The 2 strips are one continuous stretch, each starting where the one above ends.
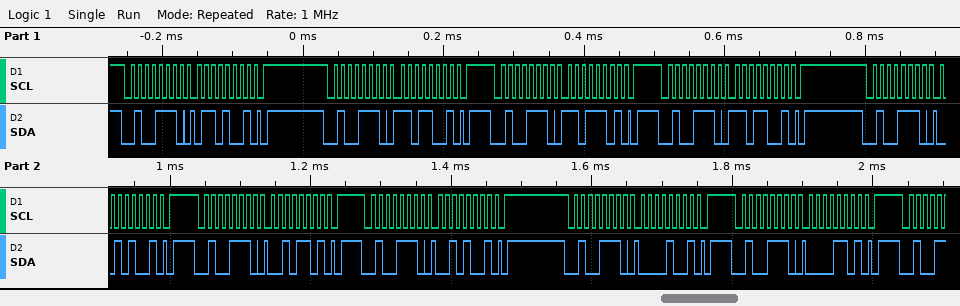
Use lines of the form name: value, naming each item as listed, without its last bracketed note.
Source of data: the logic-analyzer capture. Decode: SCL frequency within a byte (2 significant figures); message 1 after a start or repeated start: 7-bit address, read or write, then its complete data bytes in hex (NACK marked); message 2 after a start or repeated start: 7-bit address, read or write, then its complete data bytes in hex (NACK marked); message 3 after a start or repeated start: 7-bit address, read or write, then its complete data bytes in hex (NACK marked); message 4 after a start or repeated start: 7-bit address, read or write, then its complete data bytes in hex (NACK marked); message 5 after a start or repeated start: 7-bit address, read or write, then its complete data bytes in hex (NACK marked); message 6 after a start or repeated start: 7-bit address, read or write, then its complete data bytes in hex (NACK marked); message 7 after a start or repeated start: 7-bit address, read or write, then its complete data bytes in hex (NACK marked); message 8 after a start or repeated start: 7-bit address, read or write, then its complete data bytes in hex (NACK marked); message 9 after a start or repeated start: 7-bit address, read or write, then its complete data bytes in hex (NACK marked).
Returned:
SCL frequency within a byte: 100 kHz
message 1 after a start or repeated start: 7-bit address, read or write, then its complete data bytes in hex: 0x27 write: 69
message 2 after a start or repeated start: 7-bit address, read or write, then its complete data bytes in hex: 0x27 write: D9
message 3 after a start or repeated start: 7-bit address, read or write, then its complete data bytes in hex: 0x27 write: DD
message 4 after a start or repeated start: 7-bit address, read or write, then its complete data bytes in hex: 0x27 write: D9
message 5 after a start or repeated start: 7-bit address, read or write, then its complete data bytes in hex: 0x27 write: 29
message 6 after a start or repeated start: 7-bit address, read or write, then its complete data bytes in hex: 0x27 write: 2D
message 7 after a start or repeated start: 7-bit address, read or write, then its complete data bytes in hex: 0x27 write: 29
message 8 after a start or repeated start: 7-bit address, read or write, then its complete data bytes in hex: 0x27 write: 09
message 9 after a start or repeated start: 7-bit address, read or write, then its complete data bytes in hex: 0x27 write: 0D
